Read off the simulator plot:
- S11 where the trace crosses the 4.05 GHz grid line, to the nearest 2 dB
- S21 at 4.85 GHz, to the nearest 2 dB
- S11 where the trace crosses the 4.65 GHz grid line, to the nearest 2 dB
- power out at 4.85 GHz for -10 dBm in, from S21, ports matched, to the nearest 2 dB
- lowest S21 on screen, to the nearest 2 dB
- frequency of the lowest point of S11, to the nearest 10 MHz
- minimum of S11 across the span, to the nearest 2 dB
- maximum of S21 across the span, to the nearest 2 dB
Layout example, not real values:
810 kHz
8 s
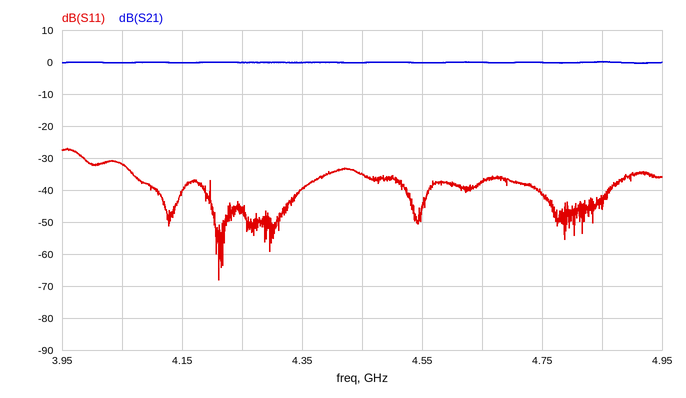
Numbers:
-32 dB
0 dB
-38 dB
-10 dBm
0 dB
4.21 GHz
-68 dB
0 dB
